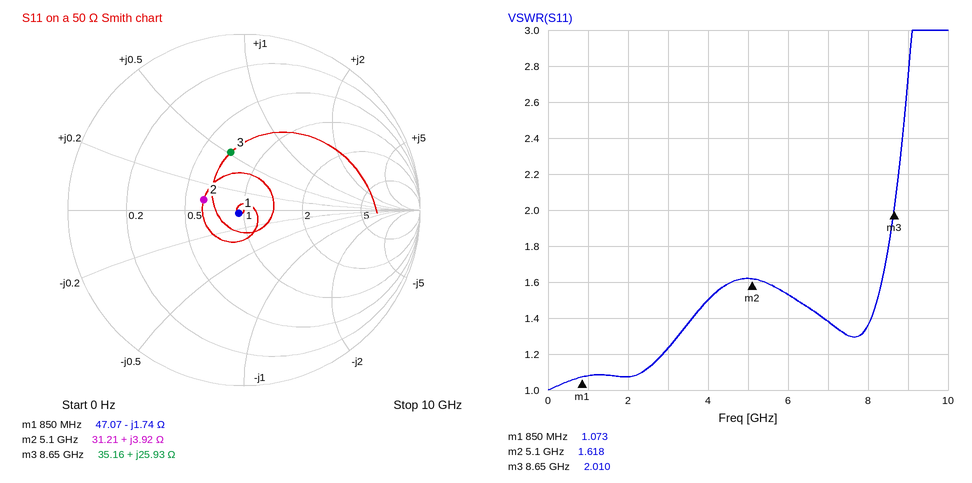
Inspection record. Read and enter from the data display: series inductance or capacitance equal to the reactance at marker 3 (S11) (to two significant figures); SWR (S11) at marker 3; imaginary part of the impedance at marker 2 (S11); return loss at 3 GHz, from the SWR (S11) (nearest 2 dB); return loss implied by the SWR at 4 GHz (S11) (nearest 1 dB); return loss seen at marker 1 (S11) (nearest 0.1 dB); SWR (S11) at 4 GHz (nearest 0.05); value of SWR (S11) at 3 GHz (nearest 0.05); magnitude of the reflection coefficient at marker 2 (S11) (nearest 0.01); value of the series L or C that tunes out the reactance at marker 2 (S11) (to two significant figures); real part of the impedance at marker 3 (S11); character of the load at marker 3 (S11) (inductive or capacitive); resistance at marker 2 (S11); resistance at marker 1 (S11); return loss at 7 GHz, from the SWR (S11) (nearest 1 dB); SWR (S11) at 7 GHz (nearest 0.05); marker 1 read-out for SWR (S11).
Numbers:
480 pH
2.010
+3.92 Ω
20 dB
14 dB
29.1 dB
1.50
1.25
0.24
8.0 pF
35.16 Ω
inductive
31.21 Ω
47.07 Ω
16 dB
1.40
1.073
